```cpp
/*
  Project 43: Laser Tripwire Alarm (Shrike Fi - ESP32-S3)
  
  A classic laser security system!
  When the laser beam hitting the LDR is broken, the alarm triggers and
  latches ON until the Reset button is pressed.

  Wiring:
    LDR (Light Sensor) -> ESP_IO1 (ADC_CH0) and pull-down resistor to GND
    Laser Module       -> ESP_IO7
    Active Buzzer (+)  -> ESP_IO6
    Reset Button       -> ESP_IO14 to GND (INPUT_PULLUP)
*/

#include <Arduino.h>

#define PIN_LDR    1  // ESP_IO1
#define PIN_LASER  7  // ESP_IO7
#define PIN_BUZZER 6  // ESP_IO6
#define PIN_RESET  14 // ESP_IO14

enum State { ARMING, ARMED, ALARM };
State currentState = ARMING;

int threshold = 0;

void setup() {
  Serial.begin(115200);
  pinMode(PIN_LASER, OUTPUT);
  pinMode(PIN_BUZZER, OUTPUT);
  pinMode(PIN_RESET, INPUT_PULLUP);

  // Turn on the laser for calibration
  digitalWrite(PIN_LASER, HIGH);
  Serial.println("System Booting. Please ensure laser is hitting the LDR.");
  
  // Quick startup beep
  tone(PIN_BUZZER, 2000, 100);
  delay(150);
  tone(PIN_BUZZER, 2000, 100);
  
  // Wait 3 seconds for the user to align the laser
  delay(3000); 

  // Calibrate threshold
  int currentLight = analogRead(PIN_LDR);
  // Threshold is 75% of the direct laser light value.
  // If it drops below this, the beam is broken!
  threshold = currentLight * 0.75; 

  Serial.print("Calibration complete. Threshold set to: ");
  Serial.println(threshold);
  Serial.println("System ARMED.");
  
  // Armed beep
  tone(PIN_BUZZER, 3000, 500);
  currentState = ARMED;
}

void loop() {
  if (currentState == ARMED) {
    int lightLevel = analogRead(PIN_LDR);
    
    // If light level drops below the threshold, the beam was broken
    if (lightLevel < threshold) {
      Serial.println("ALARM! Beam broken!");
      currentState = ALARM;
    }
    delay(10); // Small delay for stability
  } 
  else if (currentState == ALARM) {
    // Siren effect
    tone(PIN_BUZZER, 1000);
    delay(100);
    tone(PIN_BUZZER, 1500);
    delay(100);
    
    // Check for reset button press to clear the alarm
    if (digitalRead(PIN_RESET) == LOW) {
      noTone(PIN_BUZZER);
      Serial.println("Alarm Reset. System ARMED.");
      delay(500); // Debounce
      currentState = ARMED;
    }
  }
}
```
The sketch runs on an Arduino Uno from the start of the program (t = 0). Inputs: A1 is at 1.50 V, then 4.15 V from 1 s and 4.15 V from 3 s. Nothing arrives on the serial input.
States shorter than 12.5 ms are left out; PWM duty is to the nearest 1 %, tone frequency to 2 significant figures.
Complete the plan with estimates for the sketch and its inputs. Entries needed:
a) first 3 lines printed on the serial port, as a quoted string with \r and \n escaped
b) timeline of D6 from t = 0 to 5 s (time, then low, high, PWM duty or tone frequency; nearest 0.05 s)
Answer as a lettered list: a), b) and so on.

a) "System Booting. Please ensure laser is hitting the LDR.\r\nCalibration complete. Threshold set to: 636\r\nSystem ARMED.\r\n"
b) 0 s tone 2000 Hz; 0.1 s low; 0.15 s tone 2000 Hz; 0.25 s low; 3.15 s tone 3000 Hz; 3.65 s low
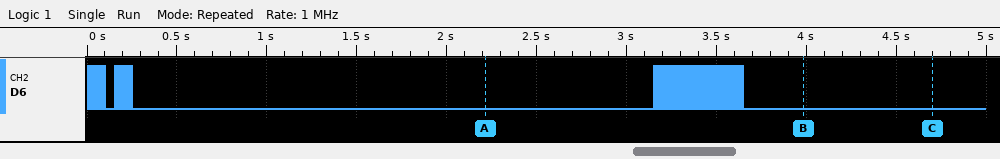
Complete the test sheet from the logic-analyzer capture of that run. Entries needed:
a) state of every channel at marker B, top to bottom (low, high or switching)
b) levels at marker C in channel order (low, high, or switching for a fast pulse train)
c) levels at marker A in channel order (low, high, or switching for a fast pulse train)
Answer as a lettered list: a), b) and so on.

a) D6 low
b) D6 low
c) D6 low
